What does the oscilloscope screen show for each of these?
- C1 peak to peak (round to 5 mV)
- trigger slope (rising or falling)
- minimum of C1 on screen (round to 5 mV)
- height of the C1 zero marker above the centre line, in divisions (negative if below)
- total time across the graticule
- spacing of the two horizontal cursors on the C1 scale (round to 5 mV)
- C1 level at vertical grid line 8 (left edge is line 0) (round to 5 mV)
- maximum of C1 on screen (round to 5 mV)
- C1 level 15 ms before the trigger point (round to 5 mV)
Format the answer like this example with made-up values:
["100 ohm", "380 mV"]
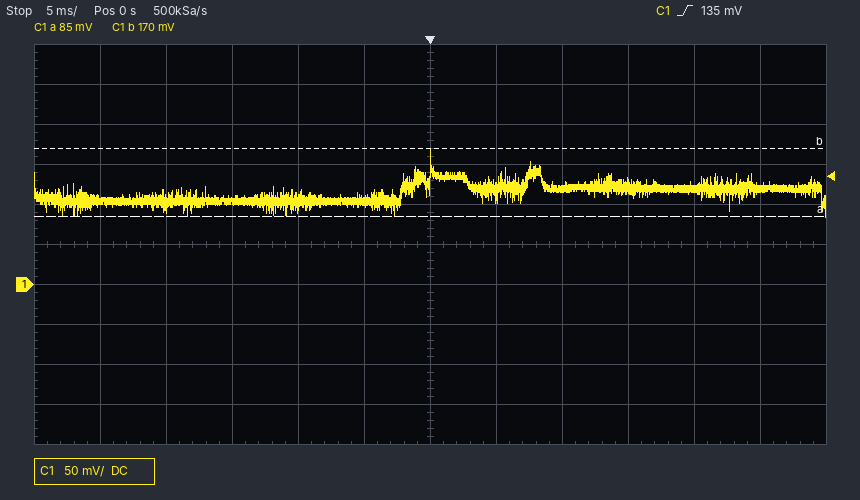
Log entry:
["85 mV", "rising", "85 mV", "-1.0 div", "60 ms", "85 mV", "120 mV", "170 mV", "105 mV"]
